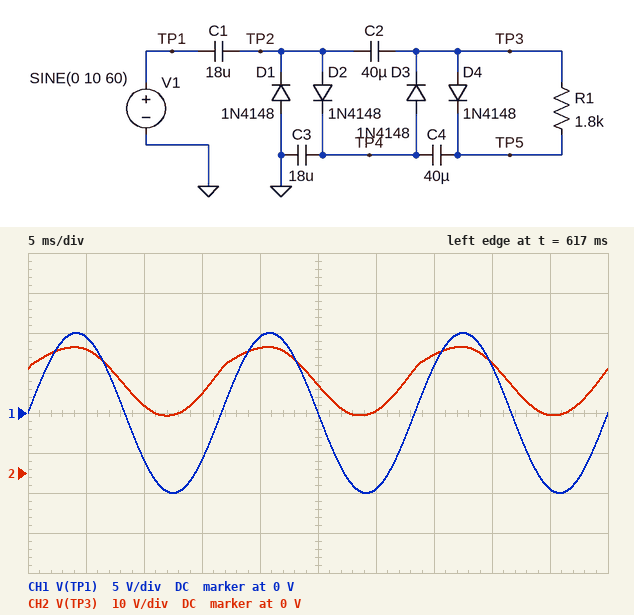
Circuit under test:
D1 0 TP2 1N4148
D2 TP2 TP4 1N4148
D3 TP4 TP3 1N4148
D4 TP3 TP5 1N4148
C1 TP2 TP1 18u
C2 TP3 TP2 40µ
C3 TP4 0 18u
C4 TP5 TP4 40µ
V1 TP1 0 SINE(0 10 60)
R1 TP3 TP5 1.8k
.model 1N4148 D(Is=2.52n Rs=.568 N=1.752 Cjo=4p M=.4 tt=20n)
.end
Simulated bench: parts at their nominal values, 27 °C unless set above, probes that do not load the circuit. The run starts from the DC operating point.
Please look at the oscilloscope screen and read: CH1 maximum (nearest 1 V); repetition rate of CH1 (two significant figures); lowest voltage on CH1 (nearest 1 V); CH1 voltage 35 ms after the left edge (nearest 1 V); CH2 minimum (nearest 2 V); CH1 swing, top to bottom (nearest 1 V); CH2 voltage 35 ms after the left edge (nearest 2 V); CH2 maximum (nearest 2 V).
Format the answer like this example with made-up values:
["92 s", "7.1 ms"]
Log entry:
["10 V", "60 Hz", "-10 V", "6 V", "14 V", "20 V", "30 V", "32 V"]
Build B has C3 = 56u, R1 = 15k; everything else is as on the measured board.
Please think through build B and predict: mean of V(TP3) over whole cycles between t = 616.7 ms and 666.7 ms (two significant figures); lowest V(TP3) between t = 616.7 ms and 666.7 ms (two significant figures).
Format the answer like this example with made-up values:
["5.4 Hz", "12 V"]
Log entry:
["27 V", "17 V"]
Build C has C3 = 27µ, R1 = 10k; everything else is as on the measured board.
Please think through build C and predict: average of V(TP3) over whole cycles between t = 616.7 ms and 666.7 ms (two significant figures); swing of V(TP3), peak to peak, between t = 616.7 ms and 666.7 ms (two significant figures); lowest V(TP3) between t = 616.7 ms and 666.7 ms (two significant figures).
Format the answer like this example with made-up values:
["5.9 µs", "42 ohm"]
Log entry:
["27 V", "19 V", "17 V"]
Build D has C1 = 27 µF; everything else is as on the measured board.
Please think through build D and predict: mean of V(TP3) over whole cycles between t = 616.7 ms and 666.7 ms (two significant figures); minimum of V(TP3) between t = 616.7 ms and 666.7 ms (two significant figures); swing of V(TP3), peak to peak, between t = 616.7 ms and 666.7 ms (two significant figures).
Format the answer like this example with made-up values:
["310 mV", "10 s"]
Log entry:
["24 V", "15 V", "18 V"]
